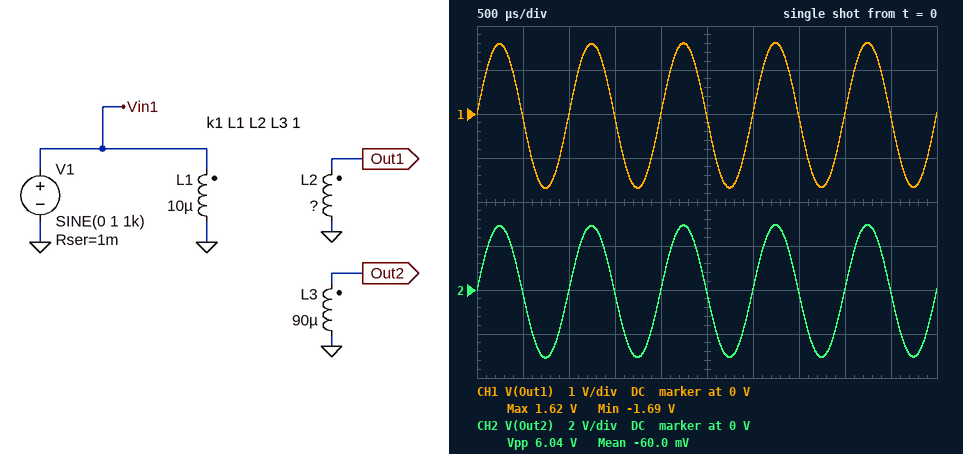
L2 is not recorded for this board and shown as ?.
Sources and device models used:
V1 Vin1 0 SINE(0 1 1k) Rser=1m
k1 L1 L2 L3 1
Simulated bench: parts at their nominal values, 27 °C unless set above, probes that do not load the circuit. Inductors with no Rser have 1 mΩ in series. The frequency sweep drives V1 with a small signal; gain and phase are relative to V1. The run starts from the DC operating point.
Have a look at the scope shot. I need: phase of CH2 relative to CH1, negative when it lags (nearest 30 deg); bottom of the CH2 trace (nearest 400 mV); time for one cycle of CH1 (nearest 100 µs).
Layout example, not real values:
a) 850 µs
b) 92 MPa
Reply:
a) 0 deg
b) -3.2 V
c) 1.0 ms
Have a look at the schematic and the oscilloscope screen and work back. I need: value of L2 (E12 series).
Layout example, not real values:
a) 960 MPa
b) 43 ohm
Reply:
a) 27 µH
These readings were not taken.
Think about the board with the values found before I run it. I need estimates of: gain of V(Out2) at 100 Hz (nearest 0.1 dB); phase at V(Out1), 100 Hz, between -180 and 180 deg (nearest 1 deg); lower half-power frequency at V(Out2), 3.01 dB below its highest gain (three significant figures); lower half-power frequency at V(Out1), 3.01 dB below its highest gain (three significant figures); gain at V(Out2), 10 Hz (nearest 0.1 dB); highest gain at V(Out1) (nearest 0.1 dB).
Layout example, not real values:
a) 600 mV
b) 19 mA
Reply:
a) 9.1 dB
b) 18 deg
c) 31.8 Hz
d) 31.8 Hz
e) -0.9 dB
f) 4.3 dB
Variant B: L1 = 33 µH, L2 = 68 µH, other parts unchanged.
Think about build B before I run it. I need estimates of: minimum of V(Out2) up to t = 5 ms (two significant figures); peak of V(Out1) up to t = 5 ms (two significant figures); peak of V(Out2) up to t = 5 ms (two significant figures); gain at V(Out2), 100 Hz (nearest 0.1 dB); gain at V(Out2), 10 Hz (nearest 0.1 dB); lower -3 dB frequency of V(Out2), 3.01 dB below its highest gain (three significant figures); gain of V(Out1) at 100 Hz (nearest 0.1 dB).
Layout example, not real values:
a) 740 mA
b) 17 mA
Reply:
a) -1.7 V
b) 1.4 V
c) 1.6 V
d) 4.3 dB
e) 1.5 dB
f) 9.65 Hz
g) 3.1 dB
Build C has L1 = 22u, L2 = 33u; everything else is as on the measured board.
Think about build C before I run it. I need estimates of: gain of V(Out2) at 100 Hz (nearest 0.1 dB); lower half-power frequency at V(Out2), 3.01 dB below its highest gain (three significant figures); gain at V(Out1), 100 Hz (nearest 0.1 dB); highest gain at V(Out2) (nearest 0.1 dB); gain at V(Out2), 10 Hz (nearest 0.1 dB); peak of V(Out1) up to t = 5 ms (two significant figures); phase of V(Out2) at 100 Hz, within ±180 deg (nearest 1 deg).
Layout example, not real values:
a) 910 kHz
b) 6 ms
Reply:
a) 6.0 dB
b) 14.5 Hz
c) 1.7 dB
d) 6.1 dB
e) 1.2 dB
f) 1.2 V
g) 8 deg
